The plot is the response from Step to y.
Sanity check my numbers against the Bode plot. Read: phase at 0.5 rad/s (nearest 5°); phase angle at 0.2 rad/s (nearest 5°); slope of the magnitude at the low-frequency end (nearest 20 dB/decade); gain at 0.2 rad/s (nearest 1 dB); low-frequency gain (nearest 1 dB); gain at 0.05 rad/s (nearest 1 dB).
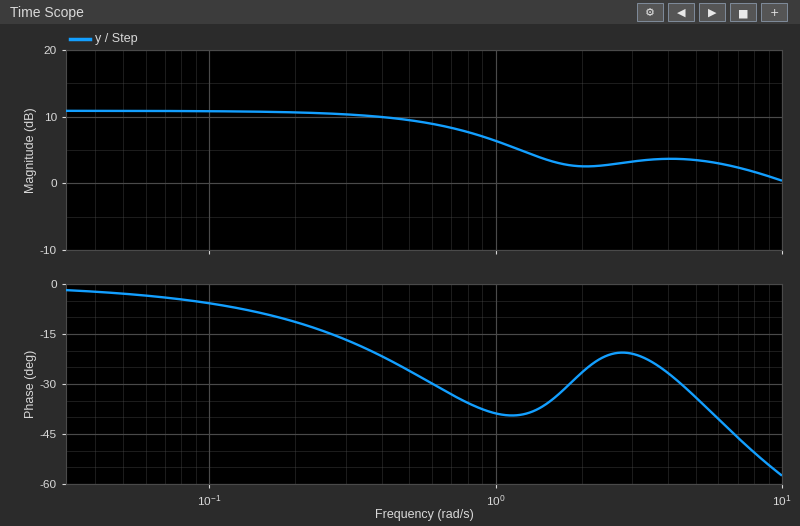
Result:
-25°
-10°
0 dB/decade
11 dB
11 dB
11 dB
